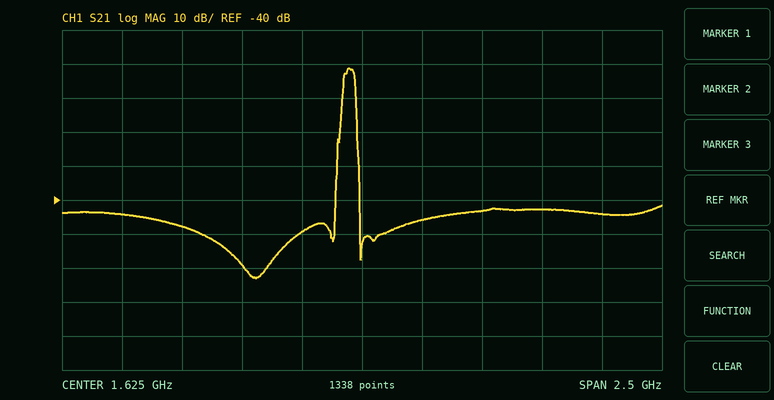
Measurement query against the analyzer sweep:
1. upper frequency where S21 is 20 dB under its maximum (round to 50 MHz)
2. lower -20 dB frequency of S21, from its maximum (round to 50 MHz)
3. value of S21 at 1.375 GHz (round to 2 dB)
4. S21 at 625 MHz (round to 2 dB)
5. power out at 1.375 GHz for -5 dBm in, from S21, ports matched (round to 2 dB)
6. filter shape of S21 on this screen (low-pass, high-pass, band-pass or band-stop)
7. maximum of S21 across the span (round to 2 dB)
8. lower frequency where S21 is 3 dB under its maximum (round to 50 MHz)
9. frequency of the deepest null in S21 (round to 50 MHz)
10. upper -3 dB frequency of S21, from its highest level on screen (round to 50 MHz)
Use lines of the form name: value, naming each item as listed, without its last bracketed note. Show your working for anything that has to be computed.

upper frequency where S21 is 20 dB under its maximum: 1.60 GHz
lower -20 dB frequency of S21, from its maximum: 1.55 GHz
value of S21 at 1.375 GHz: -50 dB
S21 at 625 MHz: -44 dB
power out at 1.375 GHz for -5 dBm in, from S21, ports matched: -5 dBm + (-50 dB) = -54 dBm
filter shape of S21 on this screen: band-pass
maximum of S21 across the span: -2 dB
lower frequency where S21 is 3 dB under its maximum: 1.55 GHz
frequency of the deepest null in S21: 1.20 GHz
upper -3 dB frequency of S21, from its highest level on screen: 1.60 GHz
